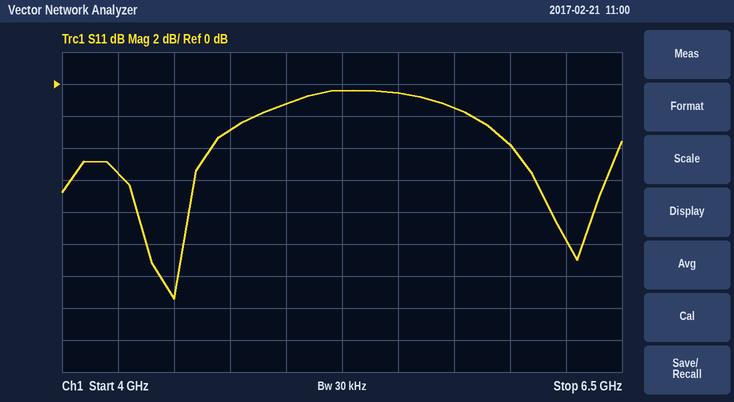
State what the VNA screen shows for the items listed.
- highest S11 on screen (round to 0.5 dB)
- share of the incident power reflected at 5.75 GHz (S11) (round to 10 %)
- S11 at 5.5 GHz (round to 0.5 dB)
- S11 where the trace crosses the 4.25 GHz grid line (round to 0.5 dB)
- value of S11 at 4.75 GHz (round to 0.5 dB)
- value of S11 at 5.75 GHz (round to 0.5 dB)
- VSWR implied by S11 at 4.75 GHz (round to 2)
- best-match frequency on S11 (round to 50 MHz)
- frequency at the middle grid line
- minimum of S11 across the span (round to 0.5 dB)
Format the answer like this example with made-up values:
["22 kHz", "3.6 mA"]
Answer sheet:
["-0.5 dB", "70 %", "-0.5 dB", "-5.5 dB", "-3.0 dB", "-1.5 dB", "6", "4.50 GHz", "5.25 GHz", "-13.5 dB"]
